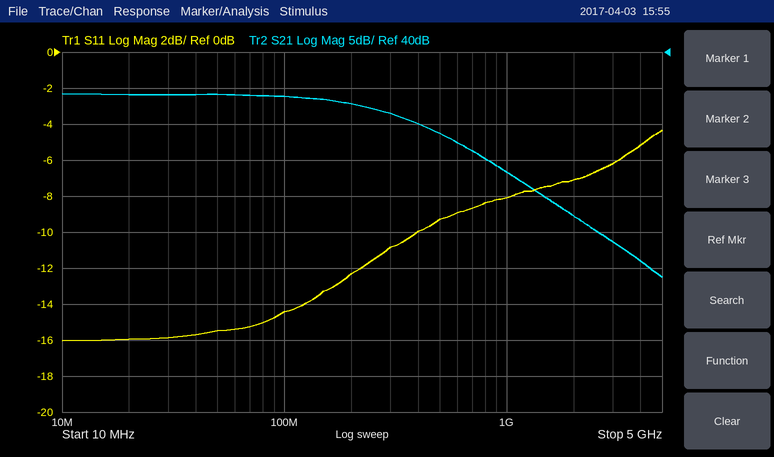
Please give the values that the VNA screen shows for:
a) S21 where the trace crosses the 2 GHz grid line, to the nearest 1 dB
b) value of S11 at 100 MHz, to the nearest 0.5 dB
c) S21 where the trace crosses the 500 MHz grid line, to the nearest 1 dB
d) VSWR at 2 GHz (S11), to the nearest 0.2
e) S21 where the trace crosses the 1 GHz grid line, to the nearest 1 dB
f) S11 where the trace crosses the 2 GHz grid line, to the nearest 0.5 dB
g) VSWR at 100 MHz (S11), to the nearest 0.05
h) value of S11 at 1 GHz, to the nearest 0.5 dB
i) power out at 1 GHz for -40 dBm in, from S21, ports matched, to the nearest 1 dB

17 dB
-14.5 dB
29 dB
2.6
23 dB
-7.0 dB
1.45
-8.0 dB
-17 dBm
